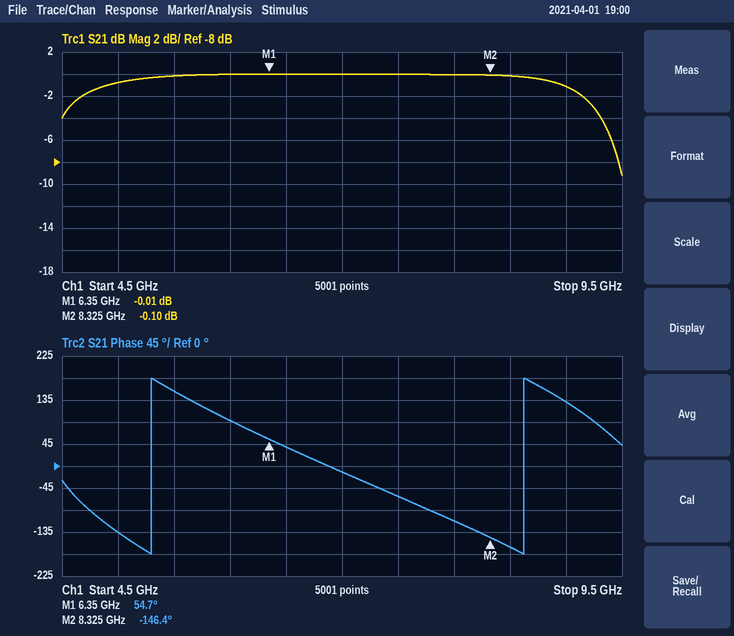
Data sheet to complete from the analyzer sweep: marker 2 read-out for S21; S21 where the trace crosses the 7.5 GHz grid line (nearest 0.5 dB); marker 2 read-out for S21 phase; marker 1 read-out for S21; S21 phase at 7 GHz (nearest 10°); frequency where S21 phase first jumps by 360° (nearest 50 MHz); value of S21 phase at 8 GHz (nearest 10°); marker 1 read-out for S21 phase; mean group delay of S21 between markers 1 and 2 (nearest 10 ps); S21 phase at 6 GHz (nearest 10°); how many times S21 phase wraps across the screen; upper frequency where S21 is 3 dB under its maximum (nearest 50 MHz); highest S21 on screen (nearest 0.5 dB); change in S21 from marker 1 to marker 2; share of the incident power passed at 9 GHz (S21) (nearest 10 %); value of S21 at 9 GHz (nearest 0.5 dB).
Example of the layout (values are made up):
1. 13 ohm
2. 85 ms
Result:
1. -0.10 dB
2. 0.0 dB
3. -146.4°
4. -0.01 dB
5. -10°
6. 5.30 GHz
7. -110°
8. 54.7°
9. 280 ps
10. 90°
11. 2
12. 9.25 GHz
13. 0.0 dB
14. -0.09 dB
15. 80 %
16. -1.0 dB
